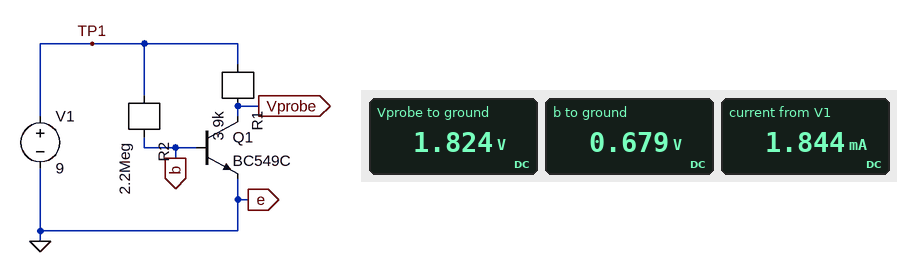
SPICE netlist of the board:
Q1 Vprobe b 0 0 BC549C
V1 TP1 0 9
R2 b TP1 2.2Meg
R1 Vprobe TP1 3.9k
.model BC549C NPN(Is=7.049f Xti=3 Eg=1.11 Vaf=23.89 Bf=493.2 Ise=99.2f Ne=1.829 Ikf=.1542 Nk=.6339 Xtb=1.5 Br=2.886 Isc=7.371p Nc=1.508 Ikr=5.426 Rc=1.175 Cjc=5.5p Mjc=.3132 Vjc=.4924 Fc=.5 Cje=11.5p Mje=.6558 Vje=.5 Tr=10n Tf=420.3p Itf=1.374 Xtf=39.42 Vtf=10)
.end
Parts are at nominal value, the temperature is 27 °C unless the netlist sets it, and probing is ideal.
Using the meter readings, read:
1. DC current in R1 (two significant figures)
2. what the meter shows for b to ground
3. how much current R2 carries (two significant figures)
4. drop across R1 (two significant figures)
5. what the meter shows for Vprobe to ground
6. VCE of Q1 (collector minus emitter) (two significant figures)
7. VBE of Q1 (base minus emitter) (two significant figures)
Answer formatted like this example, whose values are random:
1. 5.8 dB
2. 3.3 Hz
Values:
1. 1.8 mA
2. 0.679 V
3. 3.8 µA
4. 7.2 V
5. 1.824 V
6. 1.8 V
7. 680 mV
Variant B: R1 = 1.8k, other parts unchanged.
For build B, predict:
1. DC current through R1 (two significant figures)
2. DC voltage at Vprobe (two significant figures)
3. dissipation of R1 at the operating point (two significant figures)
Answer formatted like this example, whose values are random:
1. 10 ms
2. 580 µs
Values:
1. 2.1 mA
2. 5.2 V
3. 7.9 mW
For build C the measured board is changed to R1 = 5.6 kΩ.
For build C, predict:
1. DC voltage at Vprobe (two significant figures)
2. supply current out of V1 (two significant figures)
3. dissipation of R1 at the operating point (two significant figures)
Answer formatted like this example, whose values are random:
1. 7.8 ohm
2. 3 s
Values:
1. 260 mV
2. 1.6 mA
3. 14 mW
